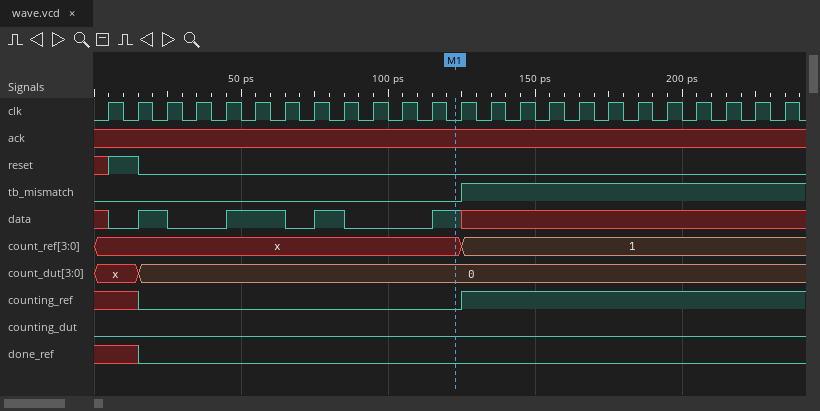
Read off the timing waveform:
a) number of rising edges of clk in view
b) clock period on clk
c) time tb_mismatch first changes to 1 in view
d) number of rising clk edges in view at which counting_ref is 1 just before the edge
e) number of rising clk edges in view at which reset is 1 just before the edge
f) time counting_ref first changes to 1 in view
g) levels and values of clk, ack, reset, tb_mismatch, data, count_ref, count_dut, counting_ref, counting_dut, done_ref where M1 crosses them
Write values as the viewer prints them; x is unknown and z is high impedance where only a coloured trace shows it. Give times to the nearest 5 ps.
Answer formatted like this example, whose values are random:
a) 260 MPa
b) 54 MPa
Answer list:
a) 24
b) 10 ps
c) 125 ps
d) 11
e) 1
f) 125 ps
g) clk=0, ack=x, reset=0, tb_mismatch=0, data=1, count_ref=x, count_dut=0, counting_ref=0, counting_dut=0, done_ref=0
